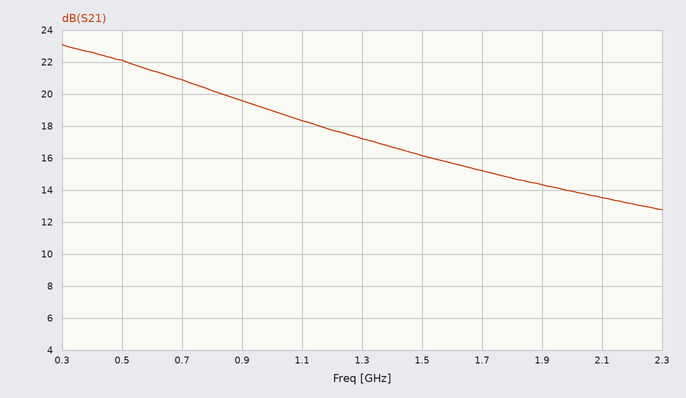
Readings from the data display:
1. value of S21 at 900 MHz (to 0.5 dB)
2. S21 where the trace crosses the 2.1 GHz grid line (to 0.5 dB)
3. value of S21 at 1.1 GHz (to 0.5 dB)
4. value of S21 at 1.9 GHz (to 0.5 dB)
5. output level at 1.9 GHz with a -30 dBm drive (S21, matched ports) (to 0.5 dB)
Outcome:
19.5 dB
13.5 dB
18.5 dB
14.5 dB
-15.5 dBm
